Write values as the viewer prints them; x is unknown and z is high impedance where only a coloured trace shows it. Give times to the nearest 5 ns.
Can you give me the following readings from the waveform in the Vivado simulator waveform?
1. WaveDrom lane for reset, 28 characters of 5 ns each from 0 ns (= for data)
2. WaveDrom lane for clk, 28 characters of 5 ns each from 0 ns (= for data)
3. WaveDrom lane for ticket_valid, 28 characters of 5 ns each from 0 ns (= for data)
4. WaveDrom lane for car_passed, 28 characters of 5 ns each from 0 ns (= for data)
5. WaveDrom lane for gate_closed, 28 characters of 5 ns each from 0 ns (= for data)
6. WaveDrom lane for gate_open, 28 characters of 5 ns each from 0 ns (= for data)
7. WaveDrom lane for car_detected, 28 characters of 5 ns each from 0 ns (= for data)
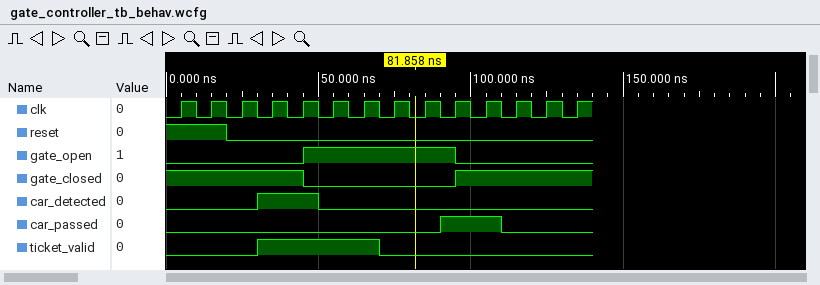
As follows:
{name: 'reset', wave: '1...0.......................'}
{name: 'clk', wave: '0101010101010101010101010101'}
{name: 'ticket_valid', wave: '0.....1.......0.............'}
{name: 'car_passed', wave: '0.................1...0.....'}
{name: 'gate_closed', wave: '1........0.........1........'}
{name: 'gate_open', wave: '0........1.........0........'}
{name: 'car_detected', wave: '0.....1...0.................'}
